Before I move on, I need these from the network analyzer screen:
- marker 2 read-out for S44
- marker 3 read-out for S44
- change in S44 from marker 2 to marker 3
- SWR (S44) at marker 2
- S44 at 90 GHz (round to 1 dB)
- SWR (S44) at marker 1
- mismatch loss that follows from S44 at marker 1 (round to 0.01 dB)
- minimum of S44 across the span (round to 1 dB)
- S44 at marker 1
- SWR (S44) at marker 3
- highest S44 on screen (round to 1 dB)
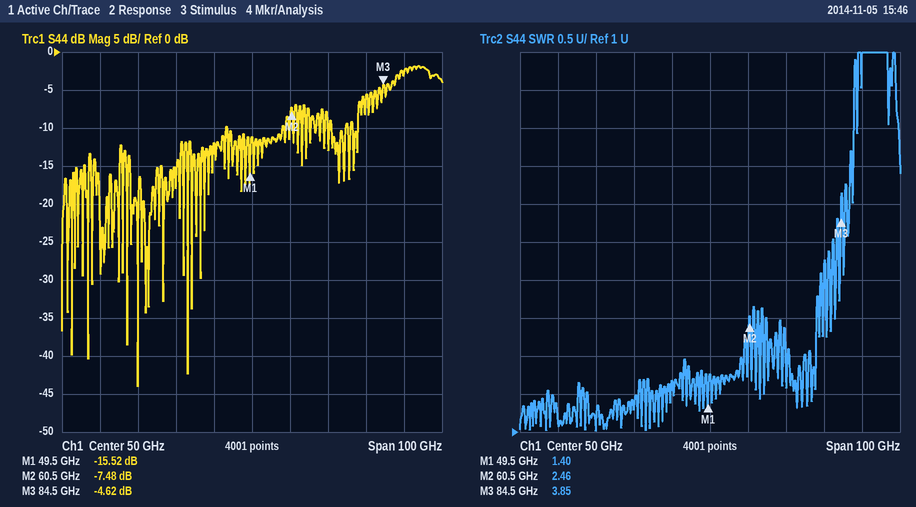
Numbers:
-7.48 dB
-4.62 dB
2.86 dB
2.46
-3 dB
1.40
0.12 dB
-44 dB
-15.52 dB
3.85
-2 dB
